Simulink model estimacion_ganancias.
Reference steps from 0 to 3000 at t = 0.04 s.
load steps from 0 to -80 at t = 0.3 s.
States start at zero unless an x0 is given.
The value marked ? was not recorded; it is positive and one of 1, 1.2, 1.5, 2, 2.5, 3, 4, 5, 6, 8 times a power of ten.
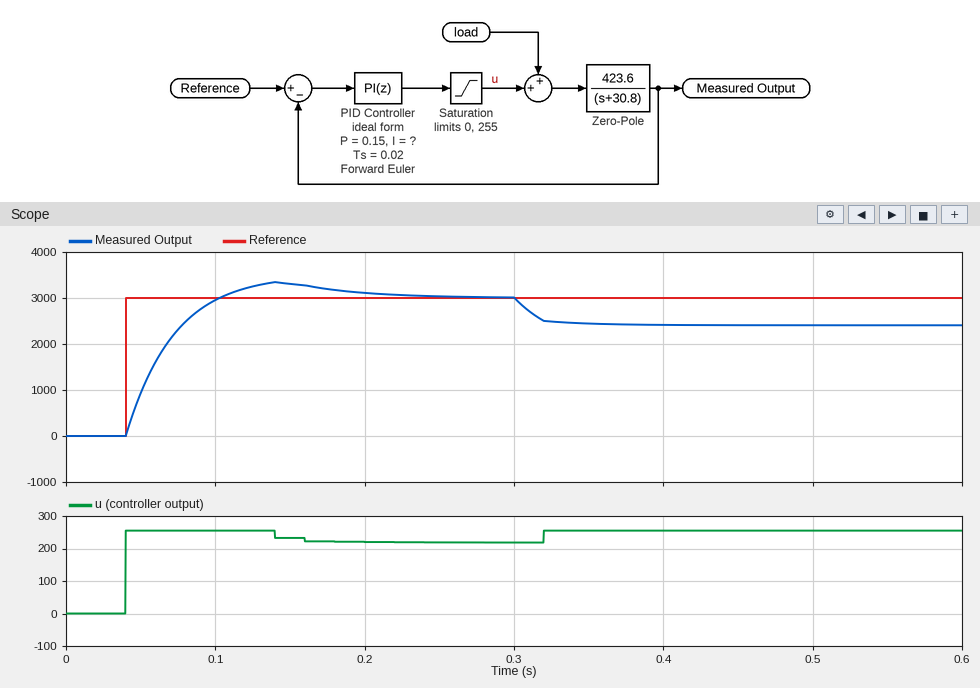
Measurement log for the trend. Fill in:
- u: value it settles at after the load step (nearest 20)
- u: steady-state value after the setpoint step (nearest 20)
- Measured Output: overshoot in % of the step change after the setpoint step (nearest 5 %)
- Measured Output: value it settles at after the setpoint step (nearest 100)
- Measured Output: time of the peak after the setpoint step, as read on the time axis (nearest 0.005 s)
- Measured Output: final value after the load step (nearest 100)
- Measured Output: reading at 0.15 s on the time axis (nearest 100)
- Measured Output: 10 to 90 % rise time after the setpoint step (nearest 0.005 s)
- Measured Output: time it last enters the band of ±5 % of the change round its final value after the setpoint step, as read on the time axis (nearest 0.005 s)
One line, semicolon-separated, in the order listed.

260; 220; 10 %; 3000; 0.140 s; 2400; 3300; 0.045 s; 0.185 s
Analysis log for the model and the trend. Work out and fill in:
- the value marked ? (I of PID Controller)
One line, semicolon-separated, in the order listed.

20
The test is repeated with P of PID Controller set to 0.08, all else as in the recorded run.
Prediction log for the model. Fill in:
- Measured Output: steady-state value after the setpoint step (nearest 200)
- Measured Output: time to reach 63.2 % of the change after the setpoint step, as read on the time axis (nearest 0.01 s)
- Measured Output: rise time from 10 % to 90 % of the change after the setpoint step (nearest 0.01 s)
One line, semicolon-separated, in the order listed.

3000; 0.07 s; 0.08 s
